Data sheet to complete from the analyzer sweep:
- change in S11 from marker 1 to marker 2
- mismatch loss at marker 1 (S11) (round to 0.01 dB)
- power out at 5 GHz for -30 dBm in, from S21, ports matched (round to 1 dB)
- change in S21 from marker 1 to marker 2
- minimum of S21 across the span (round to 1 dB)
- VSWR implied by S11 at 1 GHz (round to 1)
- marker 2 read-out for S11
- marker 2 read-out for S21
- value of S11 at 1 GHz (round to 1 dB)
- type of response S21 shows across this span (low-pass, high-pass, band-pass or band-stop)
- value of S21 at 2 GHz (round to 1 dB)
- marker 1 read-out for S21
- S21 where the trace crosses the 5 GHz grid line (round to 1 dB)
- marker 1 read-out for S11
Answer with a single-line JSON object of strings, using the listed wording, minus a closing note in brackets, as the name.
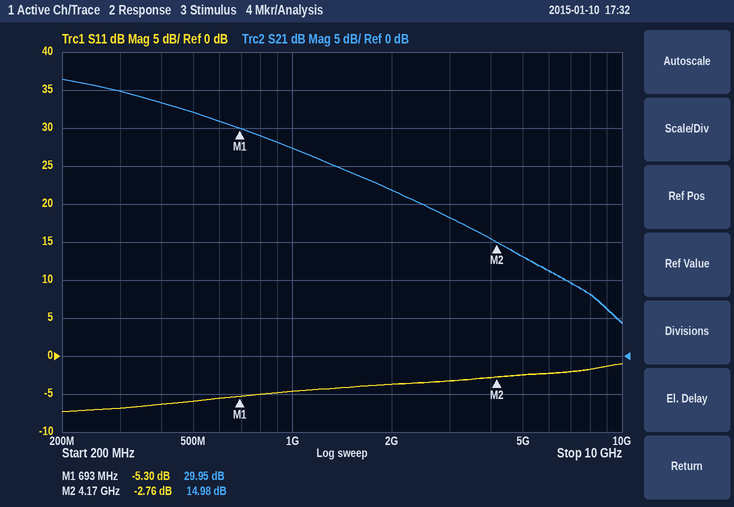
{"change in S11 from marker 1 to marker 2": "2.54 dB", "mismatch loss at marker 1 (S11)": "1.52 dB", "power out at 5 GHz for -30 dBm in, from S21, ports matched": "-17 dBm", "change in S21 from marker 1 to marker 2": "-14.97 dB", "minimum of S21 across the span": "4 dB", "VSWR implied by S11 at 1 GHz": "4", "marker 2 read-out for S11": "-2.76 dB", "marker 2 read-out for S21": "14.98 dB", "value of S11 at 1 GHz": "-5 dB", "type of response S21 shows across this span": "low-pass", "value of S21 at 2 GHz": "22 dB", "marker 1 read-out for S21": "29.95 dB", "S21 where the trace crosses the 5 GHz grid line": "13 dB", "marker 1 read-out for S11": "-5.30 dB"}
